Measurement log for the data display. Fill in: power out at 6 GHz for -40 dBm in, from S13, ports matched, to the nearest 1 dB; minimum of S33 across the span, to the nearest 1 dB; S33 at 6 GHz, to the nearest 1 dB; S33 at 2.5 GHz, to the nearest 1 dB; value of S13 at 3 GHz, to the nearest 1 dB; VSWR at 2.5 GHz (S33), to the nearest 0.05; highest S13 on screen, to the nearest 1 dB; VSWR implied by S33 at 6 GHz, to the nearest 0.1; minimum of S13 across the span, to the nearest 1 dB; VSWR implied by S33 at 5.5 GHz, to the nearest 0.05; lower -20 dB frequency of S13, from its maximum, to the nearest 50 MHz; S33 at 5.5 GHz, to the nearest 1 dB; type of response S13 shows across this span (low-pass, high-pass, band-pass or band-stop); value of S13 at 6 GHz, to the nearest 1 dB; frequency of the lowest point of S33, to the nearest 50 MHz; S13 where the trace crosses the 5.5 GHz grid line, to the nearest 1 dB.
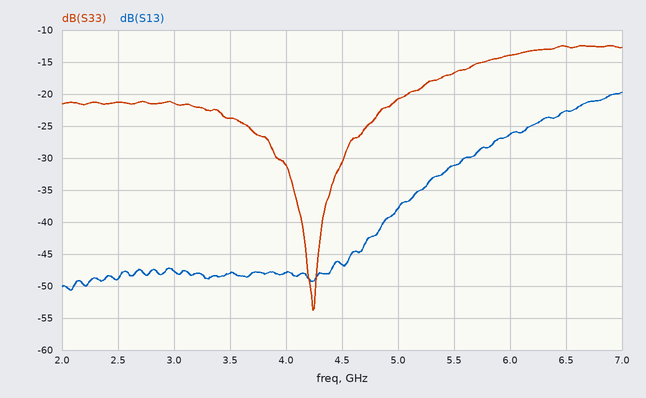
-66 dBm
-54 dB
-14 dB
-21 dB
-48 dB
1.20
-20 dB
1.5
-51 dB
1.35
4.90 GHz
-17 dB
high-pass
-26 dB
4.25 GHz
-31 dB
